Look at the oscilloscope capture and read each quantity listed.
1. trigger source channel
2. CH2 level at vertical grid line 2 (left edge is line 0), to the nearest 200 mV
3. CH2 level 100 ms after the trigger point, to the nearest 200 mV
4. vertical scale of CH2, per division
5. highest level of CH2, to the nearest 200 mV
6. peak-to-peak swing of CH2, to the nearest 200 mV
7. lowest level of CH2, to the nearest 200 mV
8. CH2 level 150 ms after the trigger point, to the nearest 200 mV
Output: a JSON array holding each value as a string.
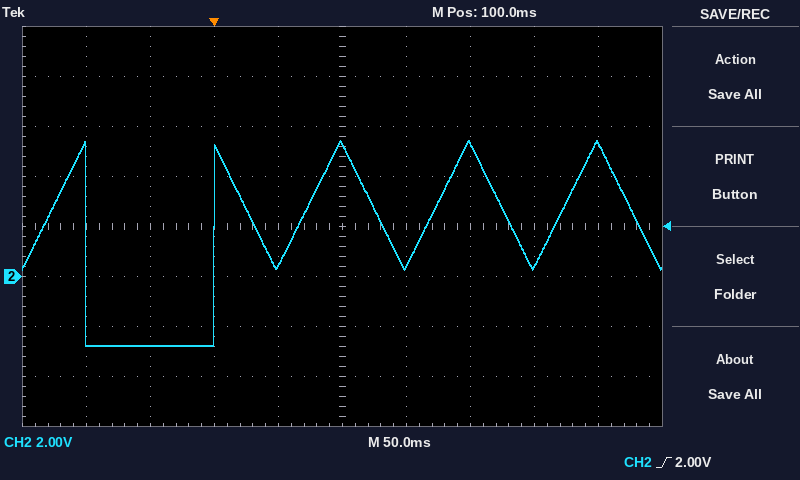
["CH2", "-2.8 V", "5.2 V", "2 V", "5.4 V", "8.2 V", "-2.8 V", "400 mV"]
